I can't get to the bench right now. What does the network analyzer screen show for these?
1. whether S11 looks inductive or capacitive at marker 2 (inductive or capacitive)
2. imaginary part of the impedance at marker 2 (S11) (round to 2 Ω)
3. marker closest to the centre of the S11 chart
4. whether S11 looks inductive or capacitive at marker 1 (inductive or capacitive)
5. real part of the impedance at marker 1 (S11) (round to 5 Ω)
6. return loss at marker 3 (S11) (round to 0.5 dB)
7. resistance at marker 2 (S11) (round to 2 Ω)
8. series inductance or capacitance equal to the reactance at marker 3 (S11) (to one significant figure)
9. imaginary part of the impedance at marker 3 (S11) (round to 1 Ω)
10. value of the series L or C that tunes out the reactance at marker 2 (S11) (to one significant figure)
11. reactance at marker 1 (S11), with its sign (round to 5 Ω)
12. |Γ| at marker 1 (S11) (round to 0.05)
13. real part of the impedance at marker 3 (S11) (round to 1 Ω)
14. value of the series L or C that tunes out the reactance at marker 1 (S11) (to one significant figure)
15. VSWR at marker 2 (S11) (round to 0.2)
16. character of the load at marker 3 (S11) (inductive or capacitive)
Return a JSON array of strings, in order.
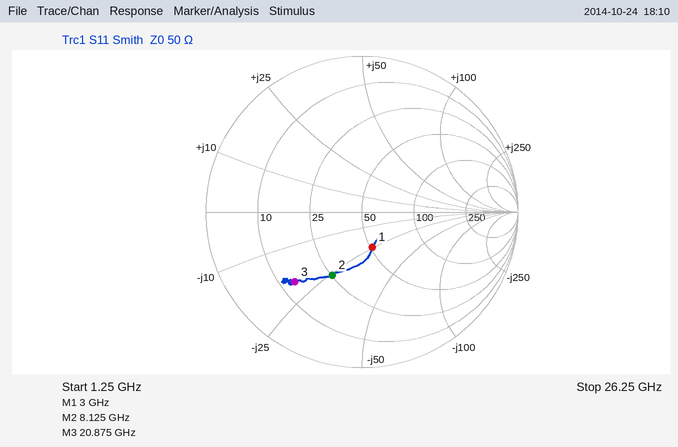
["capacitive", "-26 Ω", "marker 1", "capacitive", "50 Ω", "4.0 dB", "26 Ω", "400 fF", "-20 Ω", "500 pH", "-25 Ω", "0.25", "14 Ω", "1 nH", "2.6", "capacitive"]
